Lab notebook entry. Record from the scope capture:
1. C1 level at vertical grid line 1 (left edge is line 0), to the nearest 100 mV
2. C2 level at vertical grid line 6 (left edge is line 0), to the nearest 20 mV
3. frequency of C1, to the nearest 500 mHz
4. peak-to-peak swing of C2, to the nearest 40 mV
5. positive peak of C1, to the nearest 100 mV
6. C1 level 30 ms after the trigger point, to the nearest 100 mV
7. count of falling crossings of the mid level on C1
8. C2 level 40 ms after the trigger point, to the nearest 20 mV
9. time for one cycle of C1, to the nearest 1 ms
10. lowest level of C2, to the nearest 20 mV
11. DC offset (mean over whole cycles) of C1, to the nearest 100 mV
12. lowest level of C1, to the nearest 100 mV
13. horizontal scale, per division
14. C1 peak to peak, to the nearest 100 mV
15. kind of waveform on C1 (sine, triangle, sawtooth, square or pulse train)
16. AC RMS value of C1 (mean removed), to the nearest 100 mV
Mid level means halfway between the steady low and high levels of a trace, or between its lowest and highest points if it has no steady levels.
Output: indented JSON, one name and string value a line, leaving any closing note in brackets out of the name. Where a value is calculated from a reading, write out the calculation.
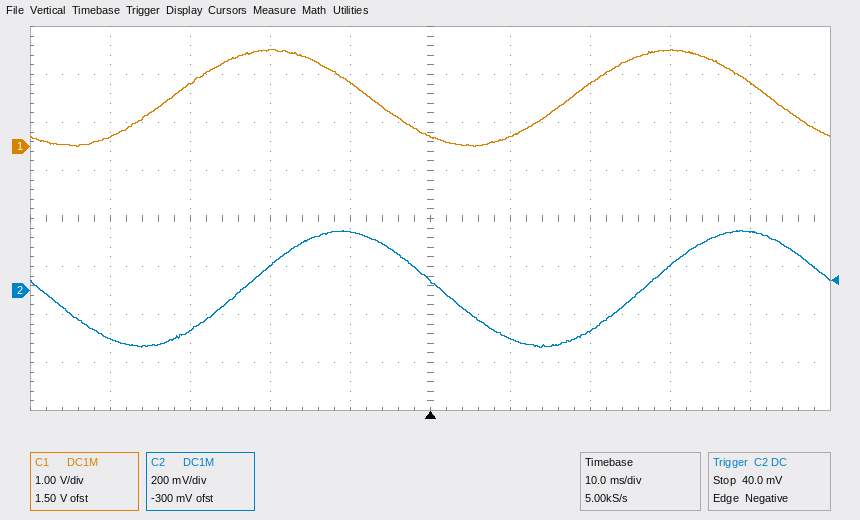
{
  "C1 level at vertical grid line 1 (left edge is line 0), to the nearest 100 mV": "200 mV",
  "C2 level at vertical grid line 6 (left edge is line 0), to the nearest 20 mV": "-200 mV",
  "frequency of C1, to the nearest 500 mHz": "1 / 50 ms ≈ 20.0 Hz",
  "peak-to-peak swing of C2, to the nearest 40 mV": "480 mV",
  "positive peak of C1, to the nearest 100 mV": "2.0 V",
  "C1 level 30 ms after the trigger point, to the nearest 100 mV": "2.0 V",
  "count of falling crossings of the mid level on C1": "2",
  "C2 level 40 ms after the trigger point, to the nearest 20 mV": "240 mV",
  "time for one cycle of C1, to the nearest 1 ms": "50 ms",
  "lowest level of C2, to the nearest 20 mV": "-240 mV",
  "DC offset (mean over whole cycles) of C1, to the nearest 100 mV": "(2.0 V + (0.0 V)) / 2 ≈ 1.0 V",
  "lowest level of C1, to the nearest 100 mV": "0.0 V",
  "horizontal scale, per division": "10 ms",
  "C1 peak to peak, to the nearest 100 mV": "2.0 V − (0.0 V) = 2.0 V",
  "kind of waveform on C1": "sine",
  "AC RMS value of C1 (mean removed), to the nearest 100 mV": "2.0 V / (2√2) ≈ 707 mV, so 700 mV to the nearest 100 mV"
}
